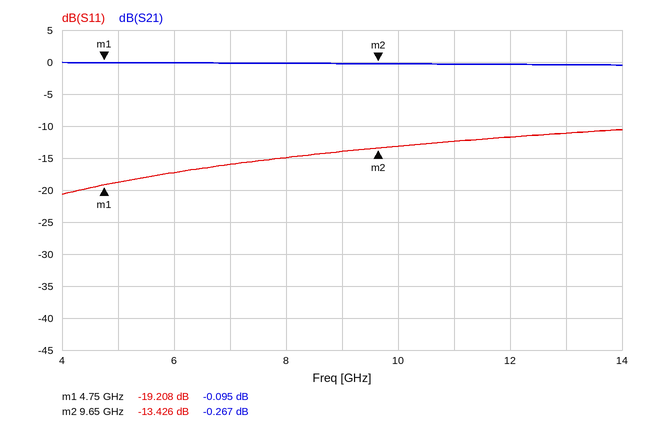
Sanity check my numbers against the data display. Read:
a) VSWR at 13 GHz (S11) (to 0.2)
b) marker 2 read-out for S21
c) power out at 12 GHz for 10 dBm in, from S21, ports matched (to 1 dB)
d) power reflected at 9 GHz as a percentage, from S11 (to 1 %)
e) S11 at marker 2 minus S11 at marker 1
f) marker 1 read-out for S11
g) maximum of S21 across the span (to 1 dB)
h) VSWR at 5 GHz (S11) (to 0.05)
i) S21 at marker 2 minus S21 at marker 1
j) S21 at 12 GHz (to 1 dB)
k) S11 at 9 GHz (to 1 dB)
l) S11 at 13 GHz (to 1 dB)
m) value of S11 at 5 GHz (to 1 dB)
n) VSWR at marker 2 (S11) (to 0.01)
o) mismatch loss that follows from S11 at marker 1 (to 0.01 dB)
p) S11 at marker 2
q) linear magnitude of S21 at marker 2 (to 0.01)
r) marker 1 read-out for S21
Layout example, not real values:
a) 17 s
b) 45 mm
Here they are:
a) 1.8
b) -0.267 dB
c) 10 dBm
d) 4 %
e) 5.782 dB
f) -19.208 dB
g) 0 dB
h) 1.25
i) -0.172 dB
j) 0 dB
k) -14 dB
l) -11 dB
m) -19 dB
n) 1.54
o) 0.05 dB
p) -13.426 dB
q) 0.97
r) -0.095 dB
